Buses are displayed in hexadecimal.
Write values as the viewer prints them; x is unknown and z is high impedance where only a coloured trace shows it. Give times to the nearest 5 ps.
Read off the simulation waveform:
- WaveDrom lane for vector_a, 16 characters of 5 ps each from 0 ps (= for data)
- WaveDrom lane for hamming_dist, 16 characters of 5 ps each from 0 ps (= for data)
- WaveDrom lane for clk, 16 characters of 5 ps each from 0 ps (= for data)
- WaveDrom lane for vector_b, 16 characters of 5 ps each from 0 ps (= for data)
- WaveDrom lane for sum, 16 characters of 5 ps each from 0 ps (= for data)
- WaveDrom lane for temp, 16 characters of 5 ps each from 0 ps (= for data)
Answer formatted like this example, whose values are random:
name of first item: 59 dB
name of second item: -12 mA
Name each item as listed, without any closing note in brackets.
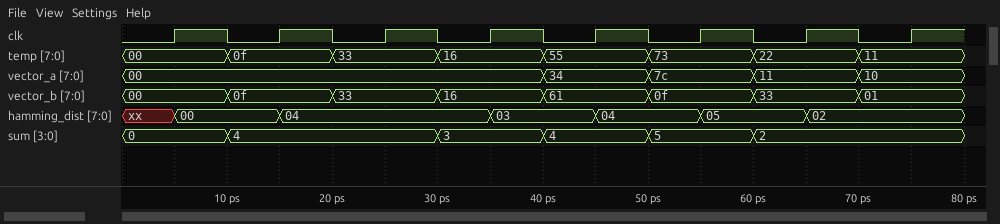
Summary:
WaveDrom lane for vector_a, 16 characters of 5 ps each from 0 ps: {name: 'vector_a', wave: '=.......=.=.=.=.', data: '00 34 7c 11 10'}
WaveDrom lane for hamming_dist, 16 characters of 5 ps each from 0 ps: {name: 'hamming_dist', wave: 'x=.=...=.=.=.=..', data: '00 04 03 04 05 02'}
WaveDrom lane for clk, 16 characters of 5 ps each from 0 ps: {name: 'clk', wave: '0101010101010101'}
WaveDrom lane for vector_b, 16 characters of 5 ps each from 0 ps: {name: 'vector_b', wave: '=.=.=.=.=.=.=.=.', data: '00 0f 33 16 61 0f 33 01'}
WaveDrom lane for sum, 16 characters of 5 ps each from 0 ps: {name: 'sum', wave: '=.=...=.=.=.=...', data: '0 4 3 4 5 2'}
WaveDrom lane for temp, 16 characters of 5 ps each from 0 ps: {name: 'temp', wave: '=.=.=.=.=.=.=.=.', data: '00 0f 33 16 55 73 22 11'}
